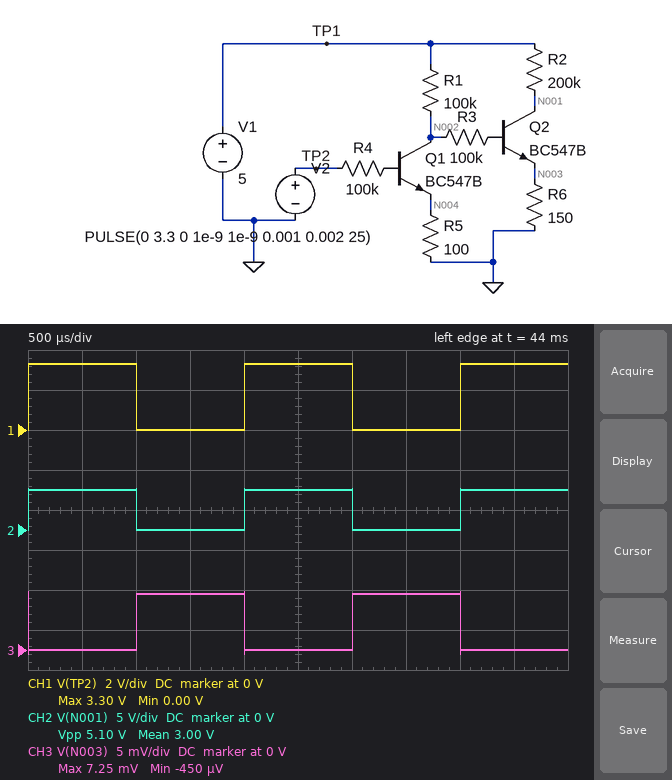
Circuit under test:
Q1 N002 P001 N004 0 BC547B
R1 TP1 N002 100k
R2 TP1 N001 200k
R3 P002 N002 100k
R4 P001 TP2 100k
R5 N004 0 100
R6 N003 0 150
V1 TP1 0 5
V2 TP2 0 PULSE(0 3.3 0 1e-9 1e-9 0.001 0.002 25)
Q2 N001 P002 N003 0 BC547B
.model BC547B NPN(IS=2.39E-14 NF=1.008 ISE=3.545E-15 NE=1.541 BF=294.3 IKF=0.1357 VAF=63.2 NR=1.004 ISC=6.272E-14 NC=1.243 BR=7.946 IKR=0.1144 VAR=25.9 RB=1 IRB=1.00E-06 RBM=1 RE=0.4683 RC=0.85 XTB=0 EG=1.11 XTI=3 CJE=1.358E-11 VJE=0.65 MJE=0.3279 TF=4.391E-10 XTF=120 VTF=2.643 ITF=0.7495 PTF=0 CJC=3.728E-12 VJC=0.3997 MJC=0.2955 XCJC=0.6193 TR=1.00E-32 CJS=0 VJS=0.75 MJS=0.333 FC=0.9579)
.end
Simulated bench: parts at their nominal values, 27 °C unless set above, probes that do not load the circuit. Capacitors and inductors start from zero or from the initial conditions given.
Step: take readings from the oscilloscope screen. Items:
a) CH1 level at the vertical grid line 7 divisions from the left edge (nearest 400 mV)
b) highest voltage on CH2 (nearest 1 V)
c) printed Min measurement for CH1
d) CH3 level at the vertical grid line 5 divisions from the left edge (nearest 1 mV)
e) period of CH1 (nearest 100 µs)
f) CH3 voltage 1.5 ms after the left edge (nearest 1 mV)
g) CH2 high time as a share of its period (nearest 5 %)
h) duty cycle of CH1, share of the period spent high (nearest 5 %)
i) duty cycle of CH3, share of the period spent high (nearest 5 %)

0 V
5 V
0.00 V
0 V
2.0 ms
7 mV
50 %
50 %
50 %
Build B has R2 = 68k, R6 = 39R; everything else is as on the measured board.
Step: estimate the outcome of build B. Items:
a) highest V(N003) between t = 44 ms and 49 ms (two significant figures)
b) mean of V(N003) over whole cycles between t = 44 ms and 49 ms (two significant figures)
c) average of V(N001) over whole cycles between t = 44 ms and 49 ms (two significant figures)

3.8 mV
1.9 mV
2.5 V
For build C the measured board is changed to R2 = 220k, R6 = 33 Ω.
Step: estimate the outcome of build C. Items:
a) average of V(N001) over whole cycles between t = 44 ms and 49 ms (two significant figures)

2.5 V
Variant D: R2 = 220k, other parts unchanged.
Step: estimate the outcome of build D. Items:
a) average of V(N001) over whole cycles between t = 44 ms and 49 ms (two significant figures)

2.5 V
